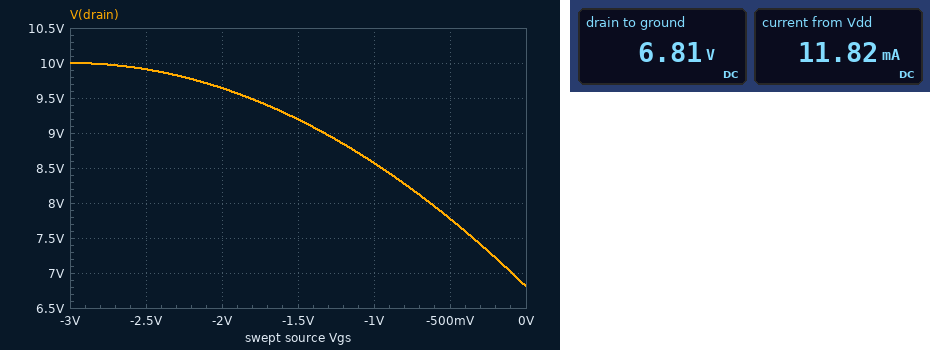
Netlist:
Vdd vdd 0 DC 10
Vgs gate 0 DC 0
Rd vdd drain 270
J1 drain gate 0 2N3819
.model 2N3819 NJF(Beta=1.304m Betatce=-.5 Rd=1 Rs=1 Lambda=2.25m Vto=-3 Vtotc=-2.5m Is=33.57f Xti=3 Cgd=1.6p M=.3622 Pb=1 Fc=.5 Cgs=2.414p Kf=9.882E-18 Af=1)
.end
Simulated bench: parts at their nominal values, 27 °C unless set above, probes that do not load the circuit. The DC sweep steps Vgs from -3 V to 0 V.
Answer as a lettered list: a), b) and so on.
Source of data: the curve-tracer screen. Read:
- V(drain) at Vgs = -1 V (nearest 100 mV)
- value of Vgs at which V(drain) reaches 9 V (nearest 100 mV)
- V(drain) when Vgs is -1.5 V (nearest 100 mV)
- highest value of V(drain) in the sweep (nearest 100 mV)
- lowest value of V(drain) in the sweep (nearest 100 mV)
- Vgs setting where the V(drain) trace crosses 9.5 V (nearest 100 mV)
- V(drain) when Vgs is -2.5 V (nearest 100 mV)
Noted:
a) 8.6 V
b) -1.3 V
c) 9.2 V
d) 10.0 V
e) 6.8 V
f) -1.8 V
g) 9.9 V
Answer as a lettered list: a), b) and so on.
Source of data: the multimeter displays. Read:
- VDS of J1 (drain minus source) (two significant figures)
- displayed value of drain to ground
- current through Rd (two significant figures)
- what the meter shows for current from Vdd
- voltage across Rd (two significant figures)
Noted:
a) 6.8 V
b) 6.81 V
c) 12 mA
d) 11.82 mA
e) 3.2 V
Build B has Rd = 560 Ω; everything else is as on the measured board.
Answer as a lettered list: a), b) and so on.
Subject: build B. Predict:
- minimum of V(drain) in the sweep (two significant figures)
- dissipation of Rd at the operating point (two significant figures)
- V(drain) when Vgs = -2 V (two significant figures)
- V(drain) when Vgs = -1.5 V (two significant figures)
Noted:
a) 3.4 V
b) 77 mW
c) 9.3 V
d) 8.3 V
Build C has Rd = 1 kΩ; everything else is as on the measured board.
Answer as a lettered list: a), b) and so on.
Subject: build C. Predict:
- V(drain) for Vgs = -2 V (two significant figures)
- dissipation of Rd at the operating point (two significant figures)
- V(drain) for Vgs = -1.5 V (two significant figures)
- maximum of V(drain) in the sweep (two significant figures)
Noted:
a) 8.7 V
b) 73 mW
c) 7.0 V
d) 10 V
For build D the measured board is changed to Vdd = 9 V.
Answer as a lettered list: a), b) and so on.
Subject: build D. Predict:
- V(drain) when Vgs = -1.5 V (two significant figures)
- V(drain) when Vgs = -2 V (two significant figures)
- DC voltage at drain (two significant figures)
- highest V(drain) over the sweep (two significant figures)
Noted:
a) 8.2 V
b) 8.6 V
c) 5.8 V
d) 9.0 V
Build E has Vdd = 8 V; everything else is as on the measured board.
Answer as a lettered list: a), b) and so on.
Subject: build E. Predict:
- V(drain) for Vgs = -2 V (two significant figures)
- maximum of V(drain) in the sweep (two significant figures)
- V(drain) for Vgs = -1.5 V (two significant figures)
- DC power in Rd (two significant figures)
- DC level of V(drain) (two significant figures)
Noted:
a) 7.6 V
b) 8.0 V
c) 7.2 V
d) 37 mW
e) 4.8 V
